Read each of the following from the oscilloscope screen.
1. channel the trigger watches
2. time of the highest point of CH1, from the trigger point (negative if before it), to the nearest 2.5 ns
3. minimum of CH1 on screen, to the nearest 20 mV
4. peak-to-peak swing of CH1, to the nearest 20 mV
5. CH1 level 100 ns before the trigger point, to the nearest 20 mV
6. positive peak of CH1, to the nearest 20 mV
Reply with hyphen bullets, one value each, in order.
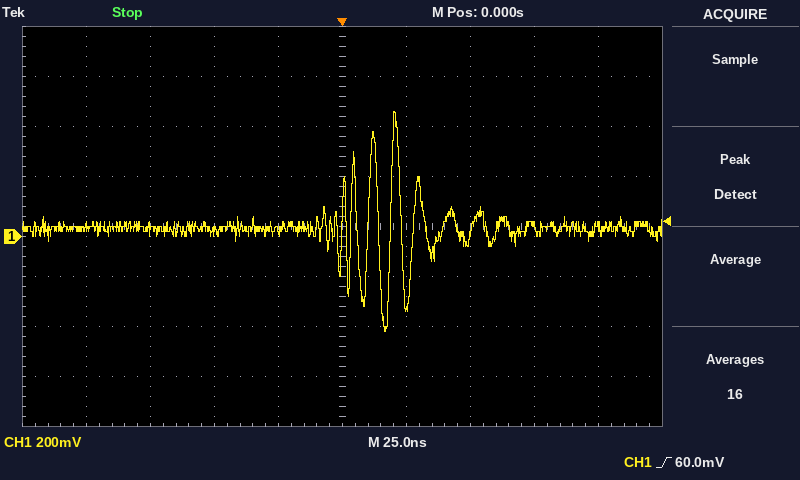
- CH1
- +20.0 ns
- -380 mV
- 880 mV
- 40 mV
- 500 mV
